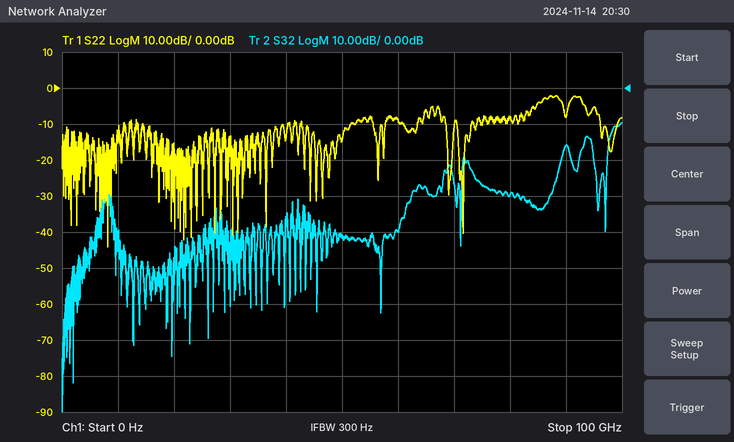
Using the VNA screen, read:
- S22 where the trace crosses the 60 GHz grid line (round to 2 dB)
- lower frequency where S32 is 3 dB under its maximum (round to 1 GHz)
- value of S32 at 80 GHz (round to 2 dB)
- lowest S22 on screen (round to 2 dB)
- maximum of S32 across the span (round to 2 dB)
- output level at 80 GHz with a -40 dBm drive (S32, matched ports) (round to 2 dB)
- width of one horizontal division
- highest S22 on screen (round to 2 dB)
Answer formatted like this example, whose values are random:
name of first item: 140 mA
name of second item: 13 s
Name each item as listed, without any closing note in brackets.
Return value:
S22 where the trace crosses the 60 GHz grid line: -8 dB
lower frequency where S32 is 3 dB under its maximum: 98 GHz
value of S32 at 80 GHz: -30 dB
lowest S22 on screen: -44 dB
maximum of S32 across the span: -10 dB
output level at 80 GHz with a -40 dBm drive (S32, matched ports): -70 dBm
width of one horizontal division: 10 GHz
highest S22 on screen: -2 dB
